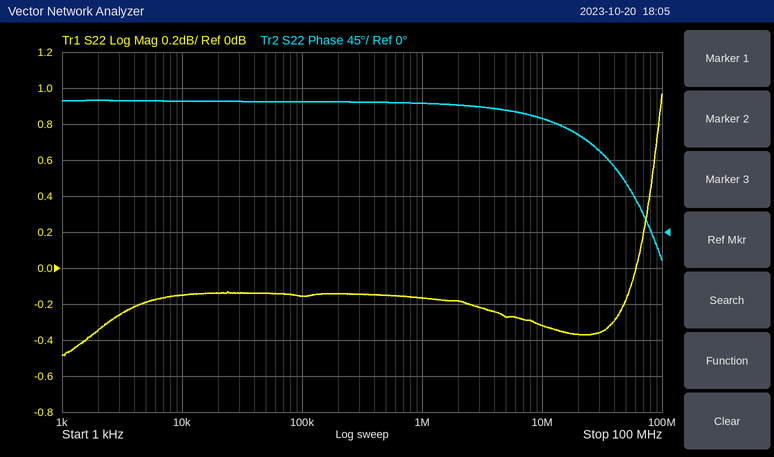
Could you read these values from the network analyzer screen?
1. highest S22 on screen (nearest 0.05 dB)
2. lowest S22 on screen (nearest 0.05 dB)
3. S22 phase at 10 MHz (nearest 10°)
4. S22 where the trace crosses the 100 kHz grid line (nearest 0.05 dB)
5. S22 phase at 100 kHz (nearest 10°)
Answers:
0.95 dB
-0.50 dB
140°
-0.15 dB
160°
